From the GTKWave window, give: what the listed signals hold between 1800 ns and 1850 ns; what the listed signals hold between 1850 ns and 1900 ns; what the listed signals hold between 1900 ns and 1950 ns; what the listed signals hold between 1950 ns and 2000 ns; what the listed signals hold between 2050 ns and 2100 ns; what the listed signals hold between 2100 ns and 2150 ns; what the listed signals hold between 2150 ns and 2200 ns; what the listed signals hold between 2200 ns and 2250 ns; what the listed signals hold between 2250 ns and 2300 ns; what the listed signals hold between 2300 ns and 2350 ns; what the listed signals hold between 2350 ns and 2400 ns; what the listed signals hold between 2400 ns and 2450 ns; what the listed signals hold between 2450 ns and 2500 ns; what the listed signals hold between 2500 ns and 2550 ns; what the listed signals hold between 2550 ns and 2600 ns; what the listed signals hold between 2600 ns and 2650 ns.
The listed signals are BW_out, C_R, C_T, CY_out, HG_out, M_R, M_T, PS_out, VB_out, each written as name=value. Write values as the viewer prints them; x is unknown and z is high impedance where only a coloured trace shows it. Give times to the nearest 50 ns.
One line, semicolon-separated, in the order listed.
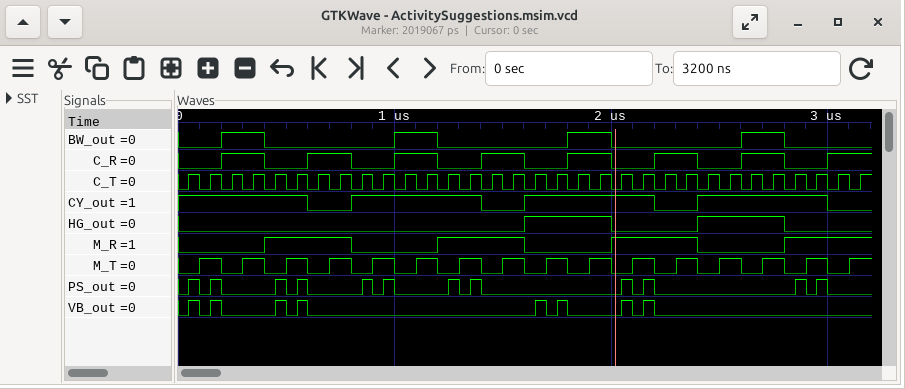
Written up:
BW_out=1, C_R=1, C_T=0, CY_out=1, HG_out=1, M_R=0, M_T=0, PS_out=0, VB_out=0; BW_out=1, C_R=1, C_T=1, CY_out=1, HG_out=1, M_R=0, M_T=0, PS_out=0, VB_out=0; BW_out=1, C_R=1, C_T=0, CY_out=1, HG_out=1, M_R=0, M_T=1, PS_out=0, VB_out=0; BW_out=1, C_R=1, C_T=1, CY_out=1, HG_out=1, M_R=0, M_T=1, PS_out=0, VB_out=0; BW_out=0, C_R=0, C_T=1, CY_out=1, HG_out=0, M_R=1, M_T=0, PS_out=1, VB_out=1; BW_out=0, C_R=0, C_T=0, CY_out=1, HG_out=0, M_R=1, M_T=1, PS_out=0, VB_out=0; BW_out=0, C_R=0, C_T=1, CY_out=1, HG_out=0, M_R=1, M_T=1, PS_out=1, VB_out=1; BW_out=0, C_R=1, C_T=0, CY_out=0, HG_out=0, M_R=1, M_T=0, PS_out=0, VB_out=0; BW_out=0, C_R=1, C_T=1, CY_out=0, HG_out=0, M_R=1, M_T=0, PS_out=0, VB_out=0; BW_out=0, C_R=1, C_T=0, CY_out=0, HG_out=0, M_R=1, M_T=1, PS_out=0, VB_out=0; BW_out=0, C_R=1, C_T=1, CY_out=0, HG_out=0, M_R=1, M_T=1, PS_out=0, VB_out=0; BW_out=0, C_R=0, C_T=0, CY_out=1, HG_out=1, M_R=0, M_T=0, PS_out=0, VB_out=0; BW_out=0, C_R=0, C_T=1, CY_out=1, HG_out=1, M_R=0, M_T=0, PS_out=0, VB_out=0; BW_out=0, C_R=0, C_T=0, CY_out=1, HG_out=1, M_R=0, M_T=1, PS_out=0, VB_out=0; BW_out=0, C_R=0, C_T=1, CY_out=1, HG_out=1, M_R=0, M_T=1, PS_out=0, VB_out=0; BW_out=1, C_R=1, C_T=0, CY_out=1, HG_out=1, M_R=0, M_T=0, PS_out=0, VB_out=0
